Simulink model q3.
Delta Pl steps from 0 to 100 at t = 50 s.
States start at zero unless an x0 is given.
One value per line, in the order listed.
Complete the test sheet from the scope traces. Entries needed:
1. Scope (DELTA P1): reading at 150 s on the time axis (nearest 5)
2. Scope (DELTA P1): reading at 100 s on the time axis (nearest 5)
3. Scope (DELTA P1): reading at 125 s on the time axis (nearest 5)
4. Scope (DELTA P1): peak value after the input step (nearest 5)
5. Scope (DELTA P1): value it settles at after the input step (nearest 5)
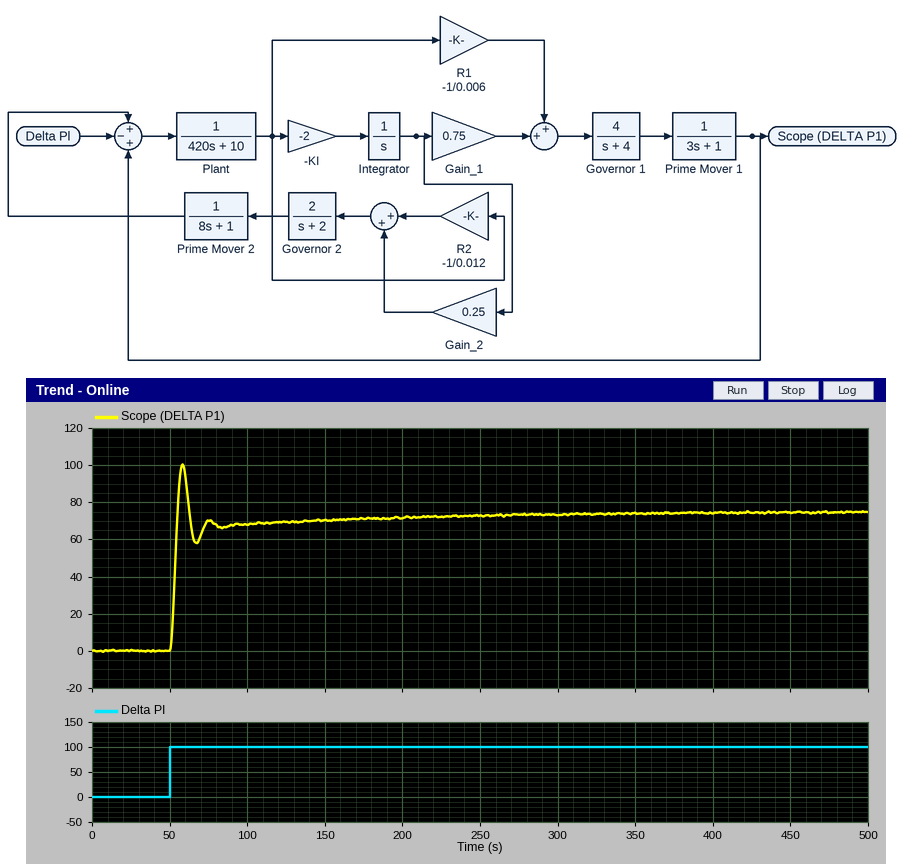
70
70
70
100
75
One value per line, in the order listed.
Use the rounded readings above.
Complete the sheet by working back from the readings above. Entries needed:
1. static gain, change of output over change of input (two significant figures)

0.75
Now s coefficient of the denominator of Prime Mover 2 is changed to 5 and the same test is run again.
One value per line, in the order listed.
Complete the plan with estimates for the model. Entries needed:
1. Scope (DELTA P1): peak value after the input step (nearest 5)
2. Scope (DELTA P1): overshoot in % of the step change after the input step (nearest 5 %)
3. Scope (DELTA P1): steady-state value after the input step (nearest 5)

95
25 %
75
